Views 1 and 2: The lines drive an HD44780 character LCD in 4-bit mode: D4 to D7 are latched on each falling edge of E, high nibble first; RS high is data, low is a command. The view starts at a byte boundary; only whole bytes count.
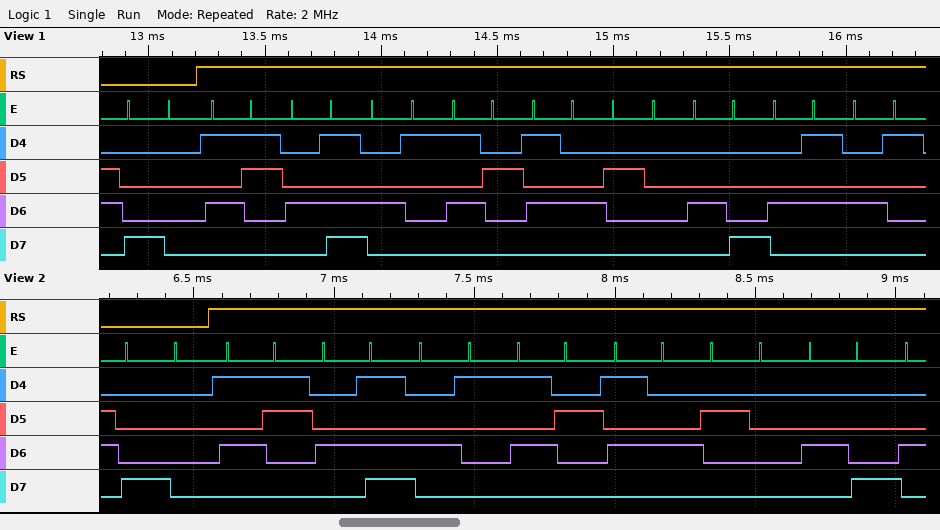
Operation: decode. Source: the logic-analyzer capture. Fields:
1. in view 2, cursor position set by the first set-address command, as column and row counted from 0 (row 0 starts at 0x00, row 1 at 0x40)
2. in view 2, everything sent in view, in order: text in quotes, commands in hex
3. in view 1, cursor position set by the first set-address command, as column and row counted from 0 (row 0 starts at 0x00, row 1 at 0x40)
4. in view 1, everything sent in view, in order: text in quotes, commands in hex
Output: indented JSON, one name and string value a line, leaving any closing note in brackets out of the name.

{
  "in view 2, cursor position set by the first set-address command, as column and row counted from 0": "column 0, row 0",
  "in view 2, everything sent in view, in order: text in quotes, commands in hex": "0x80 \"SMART H\"",
  "in view 1, cursor position set by the first set-address command, as column and row counted from 0": "column 0, row 0",
  "in view 1, everything sent in view, in order: text in quotes, commands in hex": "0x80 \"SMART HEA\""
}
